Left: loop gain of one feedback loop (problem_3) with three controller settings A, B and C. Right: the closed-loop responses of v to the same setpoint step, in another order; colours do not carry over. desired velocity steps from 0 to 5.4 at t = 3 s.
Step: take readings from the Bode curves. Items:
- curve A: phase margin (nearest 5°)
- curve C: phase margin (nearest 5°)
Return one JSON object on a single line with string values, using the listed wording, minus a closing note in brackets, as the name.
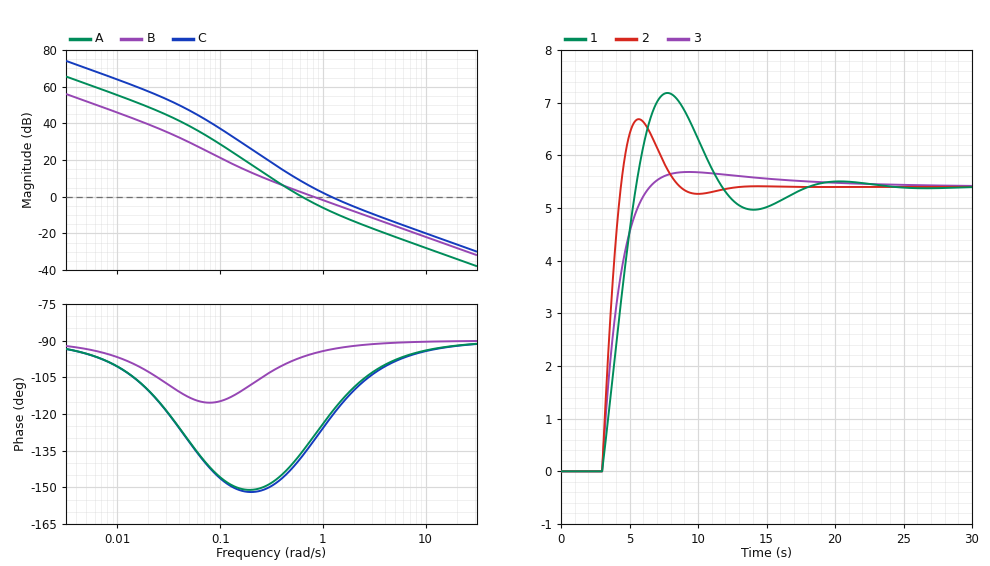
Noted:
{"curve A: phase margin": "45°", "curve C: phase margin": "60°"}
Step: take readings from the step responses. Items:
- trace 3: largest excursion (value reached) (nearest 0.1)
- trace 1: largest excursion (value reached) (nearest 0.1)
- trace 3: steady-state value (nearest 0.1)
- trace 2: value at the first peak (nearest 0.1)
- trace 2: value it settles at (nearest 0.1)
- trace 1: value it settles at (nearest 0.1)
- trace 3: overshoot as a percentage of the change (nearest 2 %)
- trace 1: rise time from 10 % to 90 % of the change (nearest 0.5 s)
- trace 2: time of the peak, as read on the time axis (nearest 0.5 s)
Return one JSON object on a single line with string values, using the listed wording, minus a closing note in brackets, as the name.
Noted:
{"trace 3: largest excursion (value reached)": "5.7", "trace 1: largest excursion (value reached)": "7.2", "trace 3: steady-state value": "5.4", "trace 2: value at the first peak": "6.7", "trace 2: value it settles at": "5.4", "trace 1: value it settles at": "5.4", "trace 3: overshoot as a percentage of the change": "6 %", "trace 1: rise time from 10 % to 90 % of the change": "2.0 s", "trace 2: time of the peak, as read on the time axis": "5.5 s"}
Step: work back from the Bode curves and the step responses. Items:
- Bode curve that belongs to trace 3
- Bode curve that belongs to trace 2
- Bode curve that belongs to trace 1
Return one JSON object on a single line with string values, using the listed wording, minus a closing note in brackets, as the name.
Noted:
{"Bode curve that belongs to trace 3": "B", "Bode curve that belongs to trace 2": "C", "Bode curve that belongs to trace 1": "A"}
